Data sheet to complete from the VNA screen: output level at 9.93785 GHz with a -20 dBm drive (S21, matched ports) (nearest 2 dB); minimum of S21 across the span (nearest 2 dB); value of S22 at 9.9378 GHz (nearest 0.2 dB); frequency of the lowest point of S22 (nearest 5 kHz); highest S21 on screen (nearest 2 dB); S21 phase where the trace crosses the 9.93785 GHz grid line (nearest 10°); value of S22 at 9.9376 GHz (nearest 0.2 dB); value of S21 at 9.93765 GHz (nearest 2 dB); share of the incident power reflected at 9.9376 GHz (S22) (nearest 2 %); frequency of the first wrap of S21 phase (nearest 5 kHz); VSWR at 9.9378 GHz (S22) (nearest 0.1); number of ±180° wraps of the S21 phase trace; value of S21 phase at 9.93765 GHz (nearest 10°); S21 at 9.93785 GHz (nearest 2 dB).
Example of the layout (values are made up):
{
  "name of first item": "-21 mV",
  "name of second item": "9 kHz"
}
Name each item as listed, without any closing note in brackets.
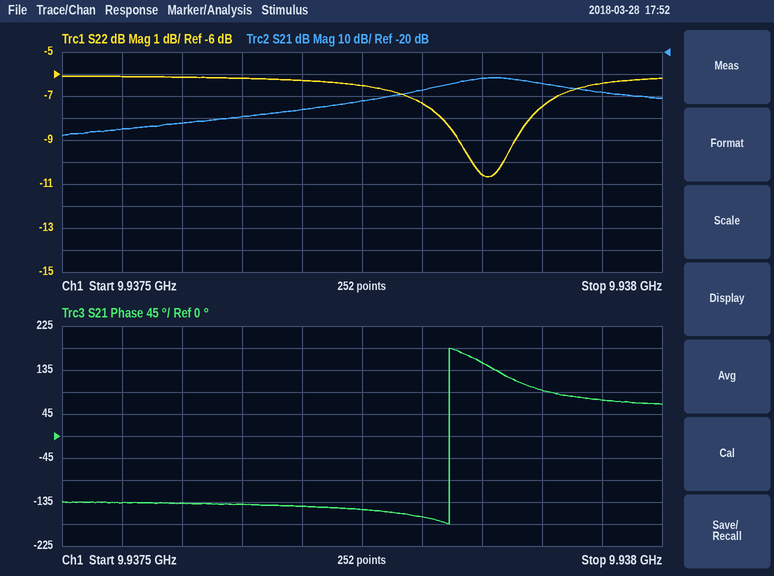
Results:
{
  "output level at 9.93785 GHz with a -20 dBm drive (S21, matched ports)": "-52 dBm",
  "minimum of S21 across the span": "-58 dB",
  "value of S22 at 9.9378 GHz": "-7.4 dB",
  "frequency of the lowest point of S22": "9.937855 GHz",
  "highest S21 on screen": "-32 dB",
  "S21 phase where the trace crosses the 9.93785 GHz grid line": "150°",
  "value of S22 at 9.9376 GHz": "-6.2 dB",
  "value of S21 at 9.93765 GHz": "-50 dB",
  "share of the incident power reflected at 9.9376 GHz (S22)": "24 %",
  "frequency of the first wrap of S21 phase": "9.937825 GHz",
  "VSWR at 9.9378 GHz (S22)": "2.5",
  "number of ±180° wraps of the S21 phase trace": "1",
  "value of S21 phase at 9.93765 GHz": "-140°",
  "S21 at 9.93785 GHz": "-32 dB"
}
